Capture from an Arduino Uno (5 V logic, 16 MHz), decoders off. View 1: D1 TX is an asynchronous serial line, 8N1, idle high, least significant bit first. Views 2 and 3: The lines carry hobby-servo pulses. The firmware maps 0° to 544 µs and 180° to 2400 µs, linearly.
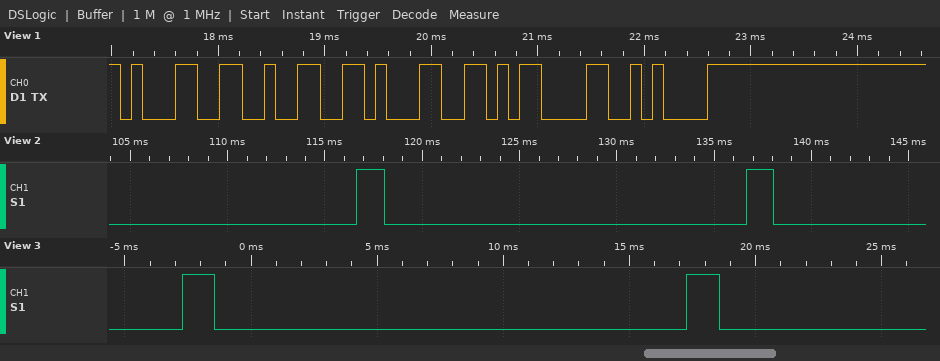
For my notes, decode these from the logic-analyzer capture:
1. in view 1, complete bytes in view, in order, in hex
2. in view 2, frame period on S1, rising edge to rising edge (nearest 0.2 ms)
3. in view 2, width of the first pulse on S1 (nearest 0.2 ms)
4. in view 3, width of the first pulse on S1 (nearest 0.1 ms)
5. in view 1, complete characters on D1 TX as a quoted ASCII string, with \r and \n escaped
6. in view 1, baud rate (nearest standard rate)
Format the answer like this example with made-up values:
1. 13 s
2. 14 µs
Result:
1. 31 32 31 0D 0A
2. 20.0 ms
3. 1.4 ms
4. 1.3 ms
5. "121\r\n"
6. 9600 baud
